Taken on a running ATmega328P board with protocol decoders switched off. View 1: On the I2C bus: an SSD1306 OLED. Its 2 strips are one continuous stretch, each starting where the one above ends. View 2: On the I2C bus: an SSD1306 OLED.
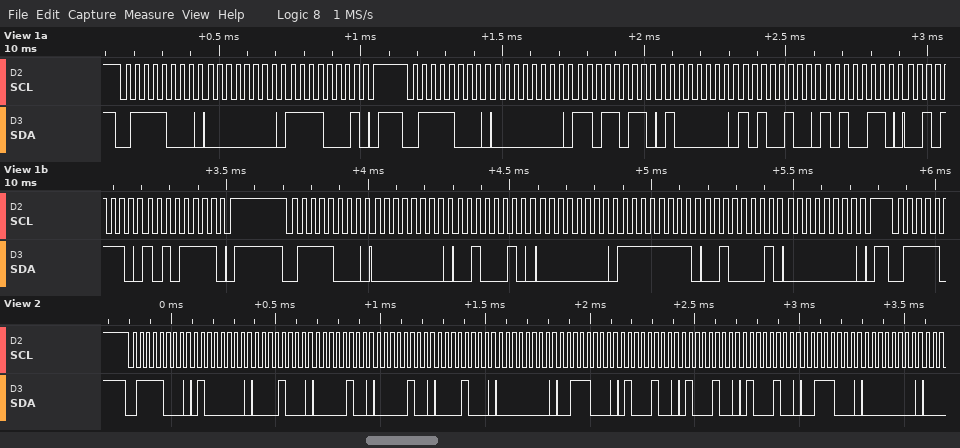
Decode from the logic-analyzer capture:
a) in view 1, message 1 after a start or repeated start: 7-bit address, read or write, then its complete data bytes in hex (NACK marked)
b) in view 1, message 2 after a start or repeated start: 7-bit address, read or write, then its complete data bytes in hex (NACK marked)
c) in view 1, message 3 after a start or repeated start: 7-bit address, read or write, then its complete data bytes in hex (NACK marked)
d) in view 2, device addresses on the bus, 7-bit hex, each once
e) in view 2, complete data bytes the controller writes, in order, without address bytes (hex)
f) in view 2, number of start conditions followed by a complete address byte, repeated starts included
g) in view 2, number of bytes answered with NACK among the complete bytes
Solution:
0x3C write: 00 F1
0x3C write: 00 DB 40 A4 A6 2E AF
0x3C write: 00 22 00 FF 21 00
0x3C
40 08 04 04 08 00 38 44 44 44 38 00
1
0
